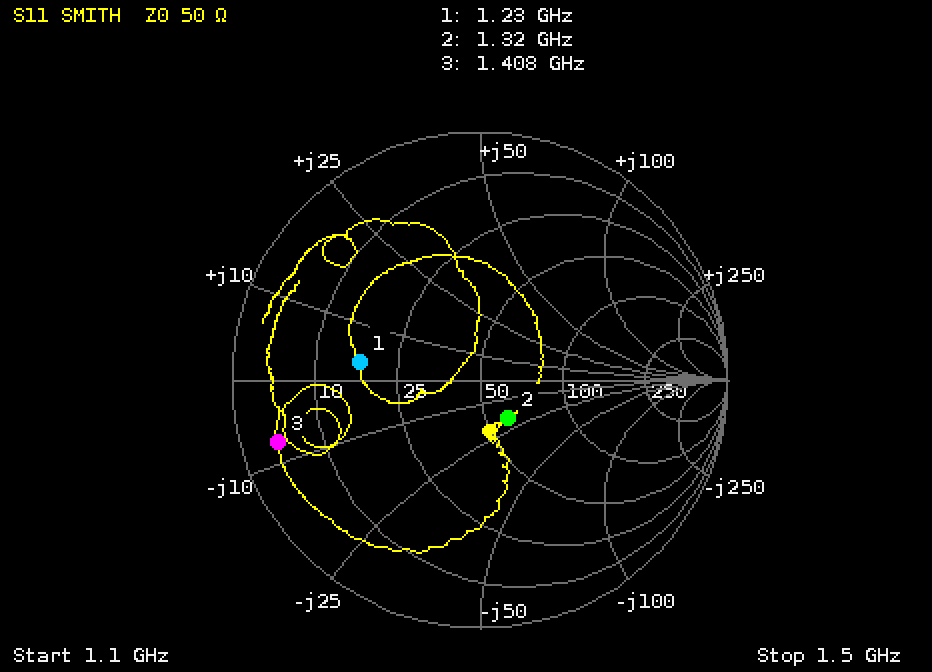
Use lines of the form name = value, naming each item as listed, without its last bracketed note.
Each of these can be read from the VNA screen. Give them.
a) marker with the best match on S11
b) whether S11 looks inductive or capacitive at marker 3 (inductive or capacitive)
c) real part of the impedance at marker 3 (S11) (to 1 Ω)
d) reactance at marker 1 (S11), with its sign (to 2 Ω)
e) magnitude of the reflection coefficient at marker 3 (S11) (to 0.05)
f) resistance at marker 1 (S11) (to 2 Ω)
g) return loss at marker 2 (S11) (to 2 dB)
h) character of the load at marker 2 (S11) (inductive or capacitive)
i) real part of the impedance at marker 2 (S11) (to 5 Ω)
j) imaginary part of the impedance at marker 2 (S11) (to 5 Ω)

marker with the best match on S11 = marker 2
whether S11 looks inductive or capacitive at marker 3 = capacitive
real part of the impedance at marker 3 (S11) = 4 Ω
reactance at marker 1 (S11), with its sign = +4 Ω
magnitude of the reflection coefficient at marker 3 (S11) = 0.85
resistance at marker 1 (S11) = 18 Ω
return loss at marker 2 (S11) = 14 dB
character of the load at marker 2 (S11) = capacitive
real part of the impedance at marker 2 (S11) = 60 Ω
imaginary part of the impedance at marker 2 (S11) = -20 Ω
